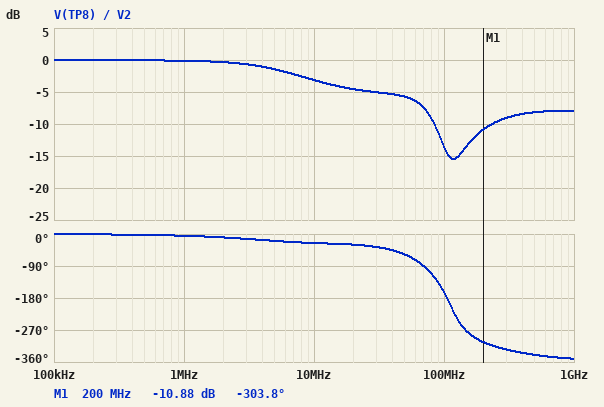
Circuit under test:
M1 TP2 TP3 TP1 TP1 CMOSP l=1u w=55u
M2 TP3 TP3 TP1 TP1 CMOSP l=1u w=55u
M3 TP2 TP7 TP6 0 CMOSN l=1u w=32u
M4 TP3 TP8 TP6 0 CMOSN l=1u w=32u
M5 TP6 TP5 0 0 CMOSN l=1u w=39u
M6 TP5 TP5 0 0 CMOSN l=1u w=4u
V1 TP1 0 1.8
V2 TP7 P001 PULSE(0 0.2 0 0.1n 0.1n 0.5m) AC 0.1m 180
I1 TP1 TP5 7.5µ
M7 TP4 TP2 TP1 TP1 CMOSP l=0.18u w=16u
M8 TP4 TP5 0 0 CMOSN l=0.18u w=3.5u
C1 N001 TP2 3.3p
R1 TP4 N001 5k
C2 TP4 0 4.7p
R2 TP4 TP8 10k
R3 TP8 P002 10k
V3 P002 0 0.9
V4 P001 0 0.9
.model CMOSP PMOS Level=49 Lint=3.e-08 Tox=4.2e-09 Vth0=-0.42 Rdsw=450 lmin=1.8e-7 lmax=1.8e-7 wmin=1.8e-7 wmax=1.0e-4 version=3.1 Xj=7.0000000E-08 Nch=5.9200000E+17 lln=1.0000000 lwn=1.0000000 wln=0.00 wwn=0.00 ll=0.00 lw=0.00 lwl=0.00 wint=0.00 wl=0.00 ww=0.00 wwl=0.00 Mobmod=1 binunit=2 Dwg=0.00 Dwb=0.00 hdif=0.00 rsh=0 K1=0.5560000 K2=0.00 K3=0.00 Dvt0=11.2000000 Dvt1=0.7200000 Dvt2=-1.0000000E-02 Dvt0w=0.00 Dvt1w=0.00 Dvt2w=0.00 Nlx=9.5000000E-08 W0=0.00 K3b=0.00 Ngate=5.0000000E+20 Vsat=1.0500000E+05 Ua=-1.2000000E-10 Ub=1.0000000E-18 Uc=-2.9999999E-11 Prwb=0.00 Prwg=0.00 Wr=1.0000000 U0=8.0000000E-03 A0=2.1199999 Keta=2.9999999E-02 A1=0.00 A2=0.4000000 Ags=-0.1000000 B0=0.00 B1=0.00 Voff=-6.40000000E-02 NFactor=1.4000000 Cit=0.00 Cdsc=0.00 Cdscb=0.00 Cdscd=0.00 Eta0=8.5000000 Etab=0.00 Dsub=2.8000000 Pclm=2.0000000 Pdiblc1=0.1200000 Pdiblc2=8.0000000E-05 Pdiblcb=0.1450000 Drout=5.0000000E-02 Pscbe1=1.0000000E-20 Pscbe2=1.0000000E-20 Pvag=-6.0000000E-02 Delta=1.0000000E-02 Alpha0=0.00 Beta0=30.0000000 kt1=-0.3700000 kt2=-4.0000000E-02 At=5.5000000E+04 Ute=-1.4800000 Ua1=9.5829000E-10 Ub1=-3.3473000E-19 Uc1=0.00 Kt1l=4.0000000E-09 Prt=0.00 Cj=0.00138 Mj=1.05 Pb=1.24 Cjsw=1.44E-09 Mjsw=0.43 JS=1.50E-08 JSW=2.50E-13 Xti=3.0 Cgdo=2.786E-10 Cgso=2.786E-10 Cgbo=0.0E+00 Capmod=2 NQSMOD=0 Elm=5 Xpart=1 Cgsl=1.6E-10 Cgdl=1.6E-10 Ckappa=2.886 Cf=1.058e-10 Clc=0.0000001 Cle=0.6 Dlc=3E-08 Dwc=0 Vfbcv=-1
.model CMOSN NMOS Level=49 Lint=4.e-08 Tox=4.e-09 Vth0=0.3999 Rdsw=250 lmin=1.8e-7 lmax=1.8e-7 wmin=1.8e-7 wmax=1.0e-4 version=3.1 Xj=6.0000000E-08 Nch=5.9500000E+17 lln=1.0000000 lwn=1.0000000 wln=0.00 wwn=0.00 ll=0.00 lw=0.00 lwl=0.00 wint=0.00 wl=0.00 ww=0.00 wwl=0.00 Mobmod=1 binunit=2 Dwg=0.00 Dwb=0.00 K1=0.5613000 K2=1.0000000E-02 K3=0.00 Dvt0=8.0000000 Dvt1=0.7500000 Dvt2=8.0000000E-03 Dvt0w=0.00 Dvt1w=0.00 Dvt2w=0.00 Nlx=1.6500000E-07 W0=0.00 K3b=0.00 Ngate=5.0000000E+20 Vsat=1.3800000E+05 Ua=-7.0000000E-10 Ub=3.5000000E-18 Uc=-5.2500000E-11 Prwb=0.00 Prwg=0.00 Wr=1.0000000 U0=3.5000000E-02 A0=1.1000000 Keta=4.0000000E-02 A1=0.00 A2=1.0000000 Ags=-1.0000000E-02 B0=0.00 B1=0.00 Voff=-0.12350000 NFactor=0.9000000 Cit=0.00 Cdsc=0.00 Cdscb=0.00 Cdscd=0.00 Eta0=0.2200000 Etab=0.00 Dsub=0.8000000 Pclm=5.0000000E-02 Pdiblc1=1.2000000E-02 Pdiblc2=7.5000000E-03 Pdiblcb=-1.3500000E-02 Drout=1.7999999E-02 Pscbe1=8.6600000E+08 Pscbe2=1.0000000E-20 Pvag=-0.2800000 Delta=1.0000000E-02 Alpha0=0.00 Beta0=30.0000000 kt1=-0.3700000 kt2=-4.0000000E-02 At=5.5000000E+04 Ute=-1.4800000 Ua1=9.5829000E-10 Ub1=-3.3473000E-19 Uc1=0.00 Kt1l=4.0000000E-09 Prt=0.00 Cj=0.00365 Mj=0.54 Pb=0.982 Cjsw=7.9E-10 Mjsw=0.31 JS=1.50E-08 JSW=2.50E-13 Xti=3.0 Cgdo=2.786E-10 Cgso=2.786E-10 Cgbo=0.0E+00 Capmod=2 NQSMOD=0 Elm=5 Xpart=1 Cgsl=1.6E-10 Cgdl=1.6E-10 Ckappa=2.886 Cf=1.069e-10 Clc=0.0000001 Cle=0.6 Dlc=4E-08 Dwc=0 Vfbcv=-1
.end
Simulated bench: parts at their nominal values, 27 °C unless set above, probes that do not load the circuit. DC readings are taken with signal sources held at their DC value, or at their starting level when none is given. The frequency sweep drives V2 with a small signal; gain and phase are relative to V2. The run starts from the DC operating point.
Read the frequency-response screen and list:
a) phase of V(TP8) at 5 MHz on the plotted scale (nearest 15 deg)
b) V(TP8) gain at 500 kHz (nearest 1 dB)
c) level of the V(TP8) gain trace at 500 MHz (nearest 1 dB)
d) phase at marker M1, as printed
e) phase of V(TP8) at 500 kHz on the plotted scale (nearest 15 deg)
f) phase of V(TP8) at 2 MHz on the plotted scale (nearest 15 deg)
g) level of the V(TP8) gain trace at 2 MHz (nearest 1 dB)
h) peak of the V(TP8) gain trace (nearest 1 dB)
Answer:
-15 deg
0 dB
-8 dB
-303.8 deg
0 deg
-15 deg
0 dB
0 dB
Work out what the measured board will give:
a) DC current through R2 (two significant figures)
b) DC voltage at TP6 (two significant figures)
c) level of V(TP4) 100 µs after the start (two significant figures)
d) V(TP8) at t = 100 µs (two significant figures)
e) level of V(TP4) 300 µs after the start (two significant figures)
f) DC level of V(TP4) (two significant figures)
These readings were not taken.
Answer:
310 nA
310 mV
1.3 V
1.1 V
1.3 V
910 mV
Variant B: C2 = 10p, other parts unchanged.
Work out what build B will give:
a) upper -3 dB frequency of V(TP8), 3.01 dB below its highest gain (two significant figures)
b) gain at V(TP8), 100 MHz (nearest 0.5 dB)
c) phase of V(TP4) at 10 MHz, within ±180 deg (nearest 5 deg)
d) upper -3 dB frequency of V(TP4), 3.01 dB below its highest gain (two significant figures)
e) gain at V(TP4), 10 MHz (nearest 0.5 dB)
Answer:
11 MHz
-17.0 dB
-30 deg
12 MHz
3.5 dB
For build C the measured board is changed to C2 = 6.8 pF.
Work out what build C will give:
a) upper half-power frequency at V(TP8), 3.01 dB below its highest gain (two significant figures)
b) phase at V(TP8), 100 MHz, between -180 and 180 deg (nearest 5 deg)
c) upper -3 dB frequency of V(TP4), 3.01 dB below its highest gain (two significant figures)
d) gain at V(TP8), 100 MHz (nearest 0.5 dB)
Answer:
10 MHz
150 deg
11 MHz
-16.5 dB
